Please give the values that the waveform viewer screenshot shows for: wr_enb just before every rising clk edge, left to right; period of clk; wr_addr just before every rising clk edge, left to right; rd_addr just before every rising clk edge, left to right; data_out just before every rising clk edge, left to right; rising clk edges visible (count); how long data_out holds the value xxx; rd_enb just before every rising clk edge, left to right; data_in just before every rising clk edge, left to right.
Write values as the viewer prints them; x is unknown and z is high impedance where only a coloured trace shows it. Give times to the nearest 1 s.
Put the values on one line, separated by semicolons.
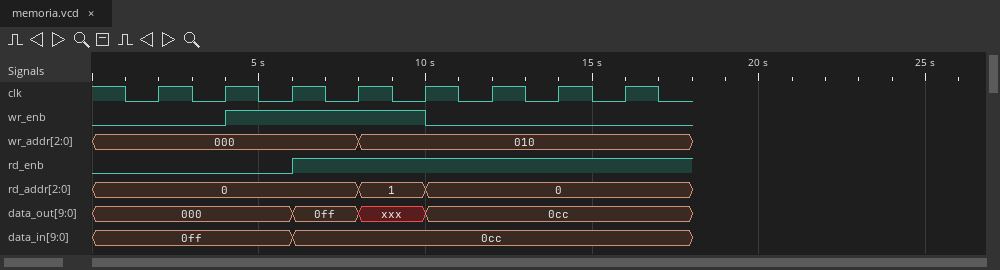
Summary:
0 0 1 1 1 0 0 0; 2 s; 000, 000, 000, 000, 010, 010, 010, 010; 0, 0, 0, 0, 1, 0, 0, 0; 000, 000, 000, 0ff, xxx, 0cc, 0cc, 0cc; 8; 2 s; 0 0 0 1 1 1 1 1; 0ff, 0ff, 0ff, 0cc, 0cc, 0cc, 0cc, 0cc
